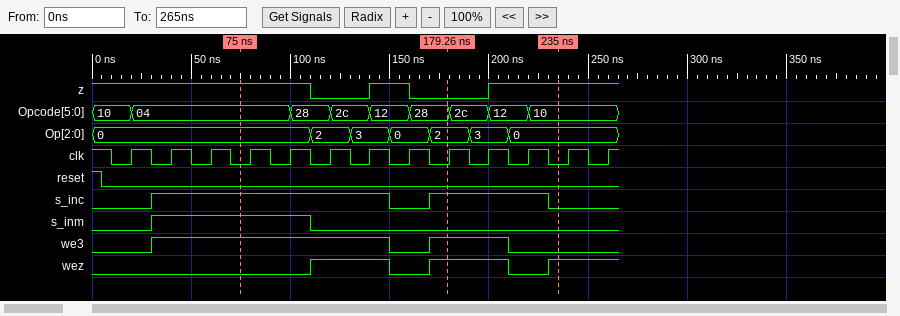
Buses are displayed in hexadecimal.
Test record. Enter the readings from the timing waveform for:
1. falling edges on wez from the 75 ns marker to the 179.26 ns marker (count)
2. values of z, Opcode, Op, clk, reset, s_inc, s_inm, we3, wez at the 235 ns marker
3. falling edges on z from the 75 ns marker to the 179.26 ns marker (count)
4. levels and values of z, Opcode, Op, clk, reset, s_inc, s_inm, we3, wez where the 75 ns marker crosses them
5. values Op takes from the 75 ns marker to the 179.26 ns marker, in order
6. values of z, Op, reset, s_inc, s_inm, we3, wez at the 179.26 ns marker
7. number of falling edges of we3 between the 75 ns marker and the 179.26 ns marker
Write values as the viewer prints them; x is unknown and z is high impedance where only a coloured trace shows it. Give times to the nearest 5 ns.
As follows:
1
z=1, Opcode=10, Op=0, clk=0, reset=0, s_inc=0, s_inm=0, we3=0, wez=1
2
z=1, Opcode=04, Op=0, clk=0, reset=0, s_inc=1, s_inm=1, we3=1, wez=0
0, 2, 3, 0, 2
z=0, Op=2, reset=0, s_inc=1, s_inm=0, we3=1, wez=1
1
